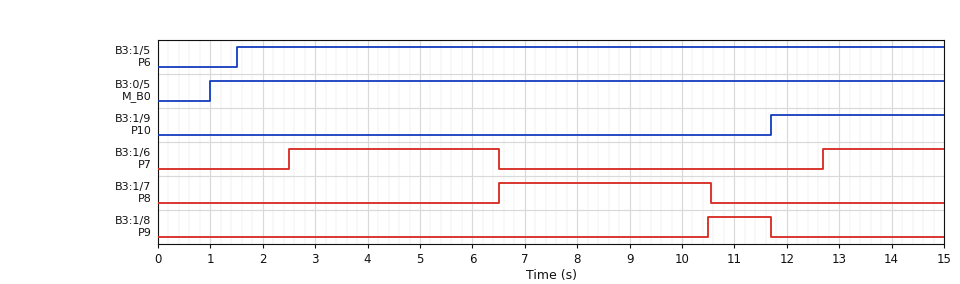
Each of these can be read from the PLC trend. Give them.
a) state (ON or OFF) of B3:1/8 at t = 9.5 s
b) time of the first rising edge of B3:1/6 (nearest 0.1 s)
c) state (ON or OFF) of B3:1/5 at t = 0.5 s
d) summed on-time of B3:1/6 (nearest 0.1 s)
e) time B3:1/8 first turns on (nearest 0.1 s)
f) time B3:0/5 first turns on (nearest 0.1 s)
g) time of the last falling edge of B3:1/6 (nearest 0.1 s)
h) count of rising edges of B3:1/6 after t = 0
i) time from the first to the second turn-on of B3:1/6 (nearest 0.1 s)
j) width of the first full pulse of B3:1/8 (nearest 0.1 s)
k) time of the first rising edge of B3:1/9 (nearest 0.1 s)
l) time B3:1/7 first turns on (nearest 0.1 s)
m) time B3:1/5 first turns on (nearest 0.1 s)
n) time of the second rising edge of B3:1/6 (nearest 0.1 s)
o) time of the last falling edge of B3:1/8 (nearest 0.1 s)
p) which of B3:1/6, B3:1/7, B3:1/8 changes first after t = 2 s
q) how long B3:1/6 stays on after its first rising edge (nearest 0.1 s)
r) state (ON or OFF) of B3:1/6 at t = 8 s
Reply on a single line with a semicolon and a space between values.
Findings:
OFF; 2.5 s; OFF; 6.3 s; 10.5 s; 1.0 s; 6.5 s; 2; 10.2 s; 1.2 s; 11.7 s; 6.5 s; 1.5 s; 12.7 s; 11.7 s; B3:1/6; 4.0 s; OFF
